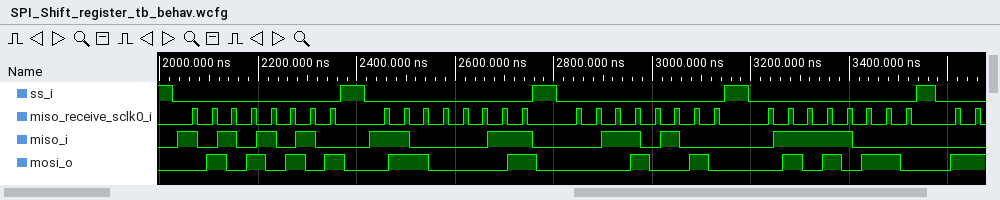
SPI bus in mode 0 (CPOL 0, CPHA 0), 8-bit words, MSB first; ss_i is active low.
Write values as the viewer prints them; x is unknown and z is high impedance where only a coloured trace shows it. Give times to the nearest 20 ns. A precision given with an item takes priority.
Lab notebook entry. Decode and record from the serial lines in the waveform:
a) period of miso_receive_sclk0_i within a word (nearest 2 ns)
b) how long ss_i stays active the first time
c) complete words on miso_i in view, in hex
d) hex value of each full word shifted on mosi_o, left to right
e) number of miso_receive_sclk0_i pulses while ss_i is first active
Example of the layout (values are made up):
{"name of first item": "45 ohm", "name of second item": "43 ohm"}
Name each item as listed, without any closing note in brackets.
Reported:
{"period of miso_receive_sclk0_i within a word": "40 ns", "how long ss_i stays active the first time": "340 ns", "complete words on miso_i in view, in hex": "AA, C3, 34, 78", "hex value of each full word shifted on mosi_o, left to right": "55, 61, 12, 56", "number of miso_receive_sclk0_i pulses while ss_i is first active": "8"}
